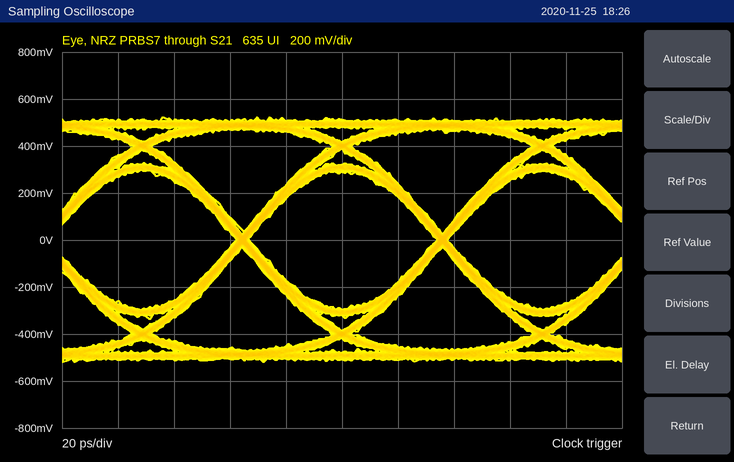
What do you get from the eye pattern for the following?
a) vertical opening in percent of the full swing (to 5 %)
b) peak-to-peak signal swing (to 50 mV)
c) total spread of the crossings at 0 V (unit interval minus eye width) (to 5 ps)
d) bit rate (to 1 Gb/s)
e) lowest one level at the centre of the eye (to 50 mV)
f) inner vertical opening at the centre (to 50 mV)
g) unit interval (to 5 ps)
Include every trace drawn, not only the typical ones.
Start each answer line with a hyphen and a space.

- 55 %
- 1.05 V
- 5 ps
- 14 Gb/s
- 300 mV
- 600 mV
- 70 ps
